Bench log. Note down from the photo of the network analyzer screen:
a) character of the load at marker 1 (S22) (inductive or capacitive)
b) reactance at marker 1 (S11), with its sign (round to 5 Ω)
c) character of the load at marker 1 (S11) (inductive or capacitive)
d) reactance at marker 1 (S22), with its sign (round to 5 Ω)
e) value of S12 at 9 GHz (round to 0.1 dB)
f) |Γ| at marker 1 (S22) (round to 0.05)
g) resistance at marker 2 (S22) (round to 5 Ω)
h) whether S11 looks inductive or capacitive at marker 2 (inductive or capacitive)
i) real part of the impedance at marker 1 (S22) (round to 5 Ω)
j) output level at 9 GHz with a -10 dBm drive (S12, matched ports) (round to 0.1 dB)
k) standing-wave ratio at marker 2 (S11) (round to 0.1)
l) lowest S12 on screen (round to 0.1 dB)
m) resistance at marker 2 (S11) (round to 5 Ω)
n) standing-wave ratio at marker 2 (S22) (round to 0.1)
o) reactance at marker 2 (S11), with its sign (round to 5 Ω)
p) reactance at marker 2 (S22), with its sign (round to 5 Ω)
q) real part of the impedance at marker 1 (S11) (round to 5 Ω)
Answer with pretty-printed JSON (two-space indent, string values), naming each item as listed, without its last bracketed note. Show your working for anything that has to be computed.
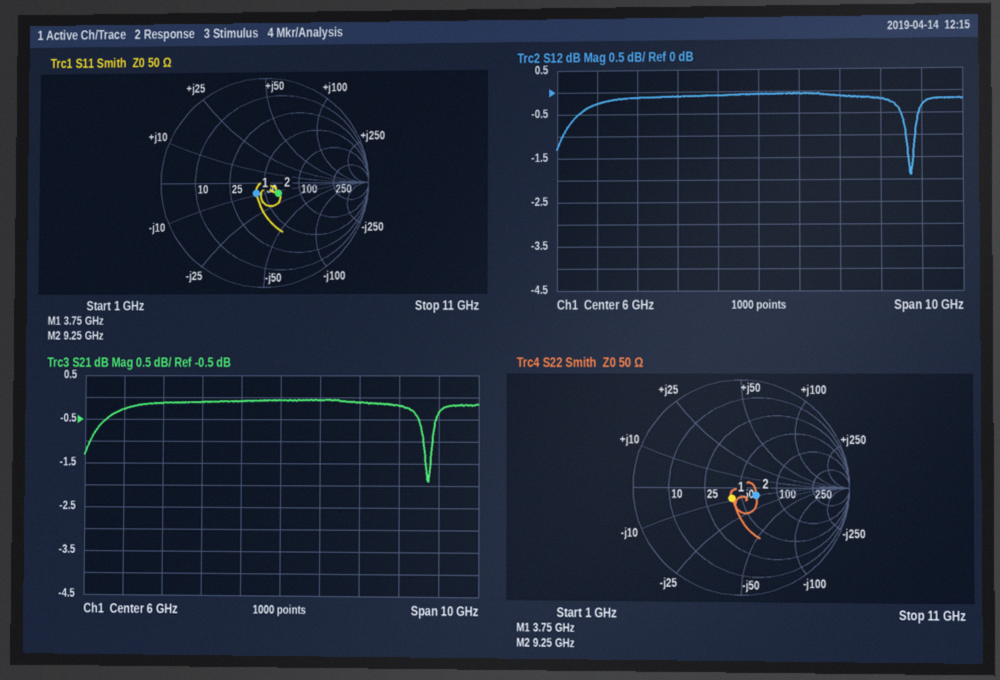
{
  "character of the load at marker 1 (S22)": "capacitive",
  "reactance at marker 1 (S11), with its sign": "-10 Ω",
  "character of the load at marker 1 (S11)": "capacitive",
  "reactance at marker 1 (S22), with its sign": "-10 Ω",
  "value of S12 at 9 GHz": "-0.2 dB",
  "|Γ| at marker 1 (S22)": "0.15",
  "resistance at marker 2 (S22)": "65 Ω",
  "whether S11 looks inductive or capacitive at marker 2": "capacitive",
  "real part of the impedance at marker 1 (S22)": "40 Ω",
  "output level at 9 GHz with a -10 dBm drive (S12, matched ports)": "-10 dBm + (-0.2 dB) = -10.2 dBm",
  "standing-wave ratio at marker 2 (S11)": "1.4",
  "lowest S12 on screen": "-1.9 dB",
  "resistance at marker 2 (S11)": "65 Ω",
  "standing-wave ratio at marker 2 (S22)": "1.4",
  "reactance at marker 2 (S11), with its sign": "-15 Ω",
  "reactance at marker 2 (S22), with its sign": "-10 Ω",
  "real part of the impedance at marker 1 (S11)": "40 Ω"
}
